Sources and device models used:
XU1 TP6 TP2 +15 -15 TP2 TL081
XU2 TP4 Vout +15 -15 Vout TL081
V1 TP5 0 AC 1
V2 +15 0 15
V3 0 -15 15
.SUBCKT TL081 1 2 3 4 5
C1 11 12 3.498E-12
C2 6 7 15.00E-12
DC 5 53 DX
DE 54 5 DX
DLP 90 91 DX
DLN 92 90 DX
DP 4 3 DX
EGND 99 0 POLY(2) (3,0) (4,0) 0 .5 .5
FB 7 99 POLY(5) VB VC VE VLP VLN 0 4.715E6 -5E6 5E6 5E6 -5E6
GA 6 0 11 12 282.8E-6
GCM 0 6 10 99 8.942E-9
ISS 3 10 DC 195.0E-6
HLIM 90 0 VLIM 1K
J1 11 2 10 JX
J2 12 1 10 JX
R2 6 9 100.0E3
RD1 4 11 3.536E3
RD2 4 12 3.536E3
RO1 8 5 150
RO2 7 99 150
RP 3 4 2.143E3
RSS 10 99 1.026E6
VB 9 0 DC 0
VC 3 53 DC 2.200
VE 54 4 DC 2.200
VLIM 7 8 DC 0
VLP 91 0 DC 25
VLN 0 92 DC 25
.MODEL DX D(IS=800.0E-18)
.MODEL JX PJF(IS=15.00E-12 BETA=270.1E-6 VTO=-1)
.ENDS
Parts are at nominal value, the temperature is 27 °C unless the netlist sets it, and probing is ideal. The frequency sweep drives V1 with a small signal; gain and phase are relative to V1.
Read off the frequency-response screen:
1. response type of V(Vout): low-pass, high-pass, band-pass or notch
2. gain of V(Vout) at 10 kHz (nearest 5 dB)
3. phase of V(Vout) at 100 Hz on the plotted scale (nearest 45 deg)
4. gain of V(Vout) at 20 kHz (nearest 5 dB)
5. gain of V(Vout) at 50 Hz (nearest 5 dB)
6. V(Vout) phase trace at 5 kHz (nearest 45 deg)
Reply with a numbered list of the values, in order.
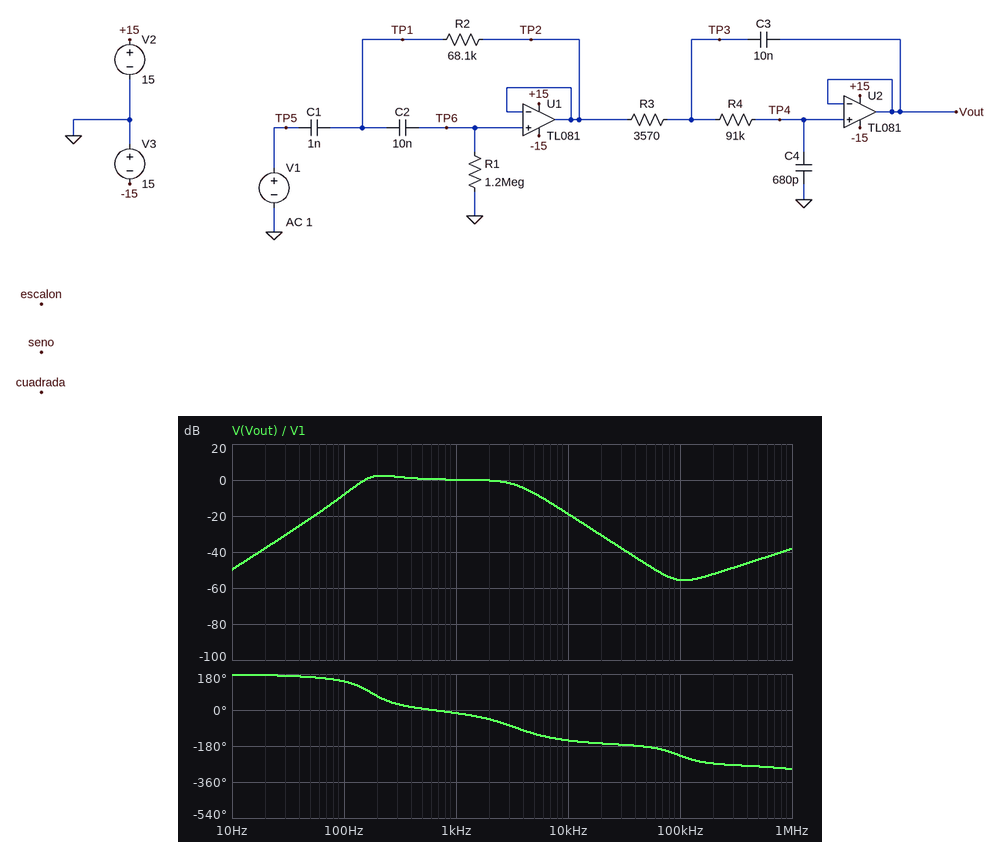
1. band-pass
2. -20 dB
3. 135 deg
4. -30 dB
5. -20 dB
6. -135 deg
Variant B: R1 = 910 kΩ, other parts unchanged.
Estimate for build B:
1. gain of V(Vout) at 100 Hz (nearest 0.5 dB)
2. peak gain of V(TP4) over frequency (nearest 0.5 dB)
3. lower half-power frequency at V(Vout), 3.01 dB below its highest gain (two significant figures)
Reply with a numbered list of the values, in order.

1. -11.0 dB
2. 1.5 dB
3. 170 Hz
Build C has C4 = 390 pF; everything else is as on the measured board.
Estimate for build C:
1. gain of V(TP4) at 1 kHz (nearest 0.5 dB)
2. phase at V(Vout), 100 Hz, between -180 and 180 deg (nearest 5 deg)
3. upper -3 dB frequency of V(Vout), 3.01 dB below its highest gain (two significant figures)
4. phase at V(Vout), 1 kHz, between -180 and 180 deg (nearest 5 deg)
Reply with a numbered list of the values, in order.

1. 0.5 dB
2. 145 deg
3. 4.6 kHz
4. -5 deg
